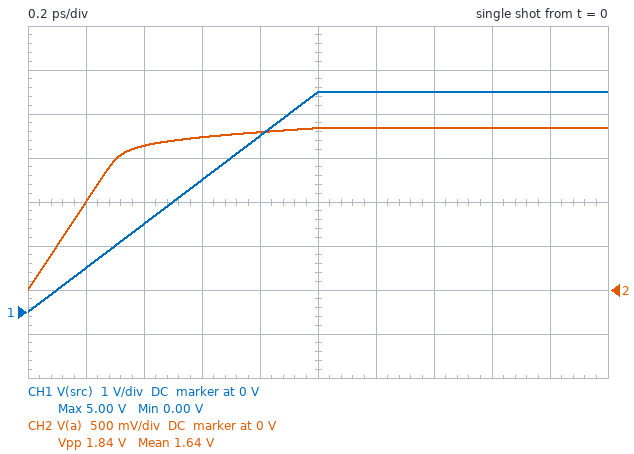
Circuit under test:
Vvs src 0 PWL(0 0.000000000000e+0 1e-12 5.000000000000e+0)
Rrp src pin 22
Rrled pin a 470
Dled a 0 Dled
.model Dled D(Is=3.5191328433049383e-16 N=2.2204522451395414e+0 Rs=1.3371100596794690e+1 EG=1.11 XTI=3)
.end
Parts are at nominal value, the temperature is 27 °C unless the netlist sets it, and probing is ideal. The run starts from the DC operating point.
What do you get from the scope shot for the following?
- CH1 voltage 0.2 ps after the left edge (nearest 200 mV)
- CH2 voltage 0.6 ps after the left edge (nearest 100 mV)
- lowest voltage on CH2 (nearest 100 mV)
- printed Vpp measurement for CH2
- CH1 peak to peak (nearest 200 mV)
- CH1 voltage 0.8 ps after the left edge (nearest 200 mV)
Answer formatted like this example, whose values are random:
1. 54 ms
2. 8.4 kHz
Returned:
1. 1.0 V
2. 1.7 V
3. 0 V
4. 1.84 V
5. 5.0 V
6. 4.0 V
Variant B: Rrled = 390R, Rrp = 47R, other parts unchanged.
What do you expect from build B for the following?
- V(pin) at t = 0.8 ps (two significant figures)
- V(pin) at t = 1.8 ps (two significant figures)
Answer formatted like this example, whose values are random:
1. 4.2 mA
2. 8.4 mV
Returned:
1. 3.8 V
2. 4.7 V
